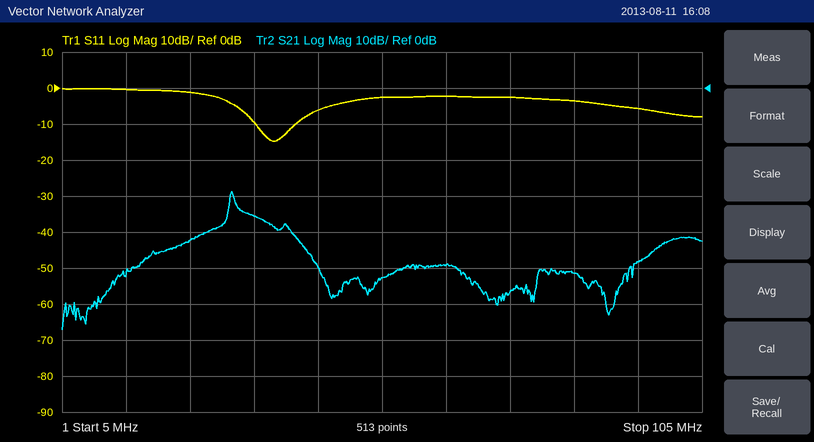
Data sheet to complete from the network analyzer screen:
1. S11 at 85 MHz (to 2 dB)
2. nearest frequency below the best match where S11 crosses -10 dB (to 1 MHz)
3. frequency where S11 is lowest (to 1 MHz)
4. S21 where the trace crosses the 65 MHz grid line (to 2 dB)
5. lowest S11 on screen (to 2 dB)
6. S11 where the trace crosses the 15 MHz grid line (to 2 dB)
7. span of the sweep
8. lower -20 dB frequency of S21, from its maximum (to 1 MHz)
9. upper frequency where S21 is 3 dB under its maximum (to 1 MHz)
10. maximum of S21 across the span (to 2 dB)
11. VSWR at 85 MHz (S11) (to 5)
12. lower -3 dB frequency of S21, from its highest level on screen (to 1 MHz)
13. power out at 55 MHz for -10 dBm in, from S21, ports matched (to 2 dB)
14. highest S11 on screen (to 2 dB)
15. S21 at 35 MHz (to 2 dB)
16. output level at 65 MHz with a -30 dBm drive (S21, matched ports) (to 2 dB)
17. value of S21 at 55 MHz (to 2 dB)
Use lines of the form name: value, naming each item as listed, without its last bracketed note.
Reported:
S11 at 85 MHz: -4 dB
nearest frequency below the best match where S11 crosses -10 dB: 35 MHz
frequency where S11 is lowest: 38 MHz
S21 where the trace crosses the 65 MHz grid line: -50 dB
lowest S11 on screen: -14 dB
S11 where the trace crosses the 15 MHz grid line: 0 dB
span of the sweep: 100 MHz
lower -20 dB frequency of S21, from its maximum: 17 MHz
upper frequency where S21 is 3 dB under its maximum: 32 MHz
maximum of S21 across the span: -28 dB
VSWR at 85 MHz (S11): 5
lower -3 dB frequency of S21, from its highest level on screen: 31 MHz
power out at 55 MHz for -10 dBm in, from S21, ports matched: -62 dBm
highest S11 on screen: 0 dB
S21 at 35 MHz: -36 dB
output level at 65 MHz with a -30 dBm drive (S21, matched ports): -80 dBm
value of S21 at 55 MHz: -52 dB
